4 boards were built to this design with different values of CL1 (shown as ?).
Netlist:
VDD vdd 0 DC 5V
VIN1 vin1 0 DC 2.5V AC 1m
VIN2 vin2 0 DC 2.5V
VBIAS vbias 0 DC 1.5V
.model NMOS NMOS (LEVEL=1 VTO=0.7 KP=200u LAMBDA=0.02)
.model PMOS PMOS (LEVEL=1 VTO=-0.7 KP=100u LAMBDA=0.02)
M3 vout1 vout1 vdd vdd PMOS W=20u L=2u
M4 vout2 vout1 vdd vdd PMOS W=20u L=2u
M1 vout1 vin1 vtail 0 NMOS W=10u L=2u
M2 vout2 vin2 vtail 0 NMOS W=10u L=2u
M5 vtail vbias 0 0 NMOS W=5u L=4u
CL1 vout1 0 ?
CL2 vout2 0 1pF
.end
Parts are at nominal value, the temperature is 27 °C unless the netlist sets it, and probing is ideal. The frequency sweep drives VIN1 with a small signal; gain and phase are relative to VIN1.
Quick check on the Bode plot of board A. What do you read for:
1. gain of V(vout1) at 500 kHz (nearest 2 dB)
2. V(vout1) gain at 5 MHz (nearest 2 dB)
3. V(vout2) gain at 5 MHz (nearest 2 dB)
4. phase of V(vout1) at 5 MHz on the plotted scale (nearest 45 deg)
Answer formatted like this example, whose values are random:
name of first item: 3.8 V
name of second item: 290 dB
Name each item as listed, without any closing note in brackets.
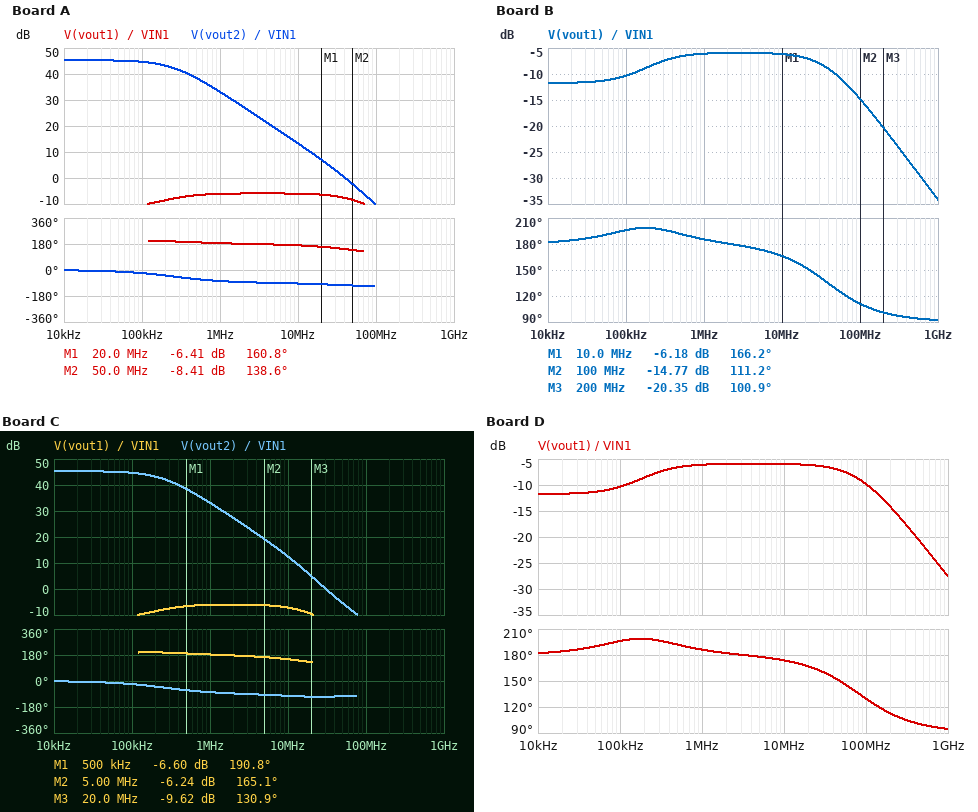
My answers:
gain of V(vout1) at 500 kHz: -6 dB
V(vout1) gain at 5 MHz: -6 dB
V(vout2) gain at 5 MHz: 20 dB
phase of V(vout1) at 5 MHz on the plotted scale: 180 deg
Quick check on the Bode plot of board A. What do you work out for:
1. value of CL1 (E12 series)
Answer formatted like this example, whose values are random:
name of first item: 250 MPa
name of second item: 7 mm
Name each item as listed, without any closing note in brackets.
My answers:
value of CL1: 820 fF
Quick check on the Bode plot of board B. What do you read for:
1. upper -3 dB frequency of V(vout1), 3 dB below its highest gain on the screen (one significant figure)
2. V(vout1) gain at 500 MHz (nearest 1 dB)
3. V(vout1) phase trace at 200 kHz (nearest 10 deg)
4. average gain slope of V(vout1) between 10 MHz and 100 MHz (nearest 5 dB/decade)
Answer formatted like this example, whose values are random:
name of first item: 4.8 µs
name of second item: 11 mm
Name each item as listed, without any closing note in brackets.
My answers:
upper -3 dB frequency of V(vout1), 3 dB below its highest gain on the screen: 40 MHz
V(vout1) gain at 500 MHz: -28 dB
V(vout1) phase trace at 200 kHz: 200 deg
average gain slope of V(vout1) between 10 MHz and 100 MHz: -10 dB/decade
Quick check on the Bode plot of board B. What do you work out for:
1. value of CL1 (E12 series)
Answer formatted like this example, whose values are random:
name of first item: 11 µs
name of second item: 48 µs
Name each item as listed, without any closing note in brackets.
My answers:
value of CL1: 1.2 pF
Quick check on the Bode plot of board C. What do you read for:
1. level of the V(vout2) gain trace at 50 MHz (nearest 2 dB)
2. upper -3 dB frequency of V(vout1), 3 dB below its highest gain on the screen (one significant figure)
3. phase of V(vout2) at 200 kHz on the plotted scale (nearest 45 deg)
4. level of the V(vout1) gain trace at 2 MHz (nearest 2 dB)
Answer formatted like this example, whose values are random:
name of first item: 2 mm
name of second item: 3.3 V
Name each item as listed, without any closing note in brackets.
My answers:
level of the V(vout2) gain trace at 50 MHz: -6 dB
upper -3 dB frequency of V(vout1), 3 dB below its highest gain on the screen: 20 MHz
phase of V(vout2) at 200 kHz on the plotted scale: -45 deg
level of the V(vout1) gain trace at 2 MHz: -6 dB
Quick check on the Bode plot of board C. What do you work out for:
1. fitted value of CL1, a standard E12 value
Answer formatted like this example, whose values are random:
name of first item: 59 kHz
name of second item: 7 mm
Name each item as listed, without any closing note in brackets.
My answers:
fitted value of CL1, a standard E12 value: 2.7 pF
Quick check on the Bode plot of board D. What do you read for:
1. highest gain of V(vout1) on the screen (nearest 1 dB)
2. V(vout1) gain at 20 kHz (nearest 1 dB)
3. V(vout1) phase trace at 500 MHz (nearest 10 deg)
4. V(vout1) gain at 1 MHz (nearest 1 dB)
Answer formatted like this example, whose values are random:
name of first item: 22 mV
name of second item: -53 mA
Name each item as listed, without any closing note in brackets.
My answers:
highest gain of V(vout1) on the screen: -6 dB
V(vout1) gain at 20 kHz: -12 dB
V(vout1) phase trace at 500 MHz: 100 deg
V(vout1) gain at 1 MHz: -6 dB
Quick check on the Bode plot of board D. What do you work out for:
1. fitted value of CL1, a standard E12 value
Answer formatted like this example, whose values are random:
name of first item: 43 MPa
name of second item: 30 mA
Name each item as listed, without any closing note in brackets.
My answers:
fitted value of CL1, a standard E12 value: 560 fF
